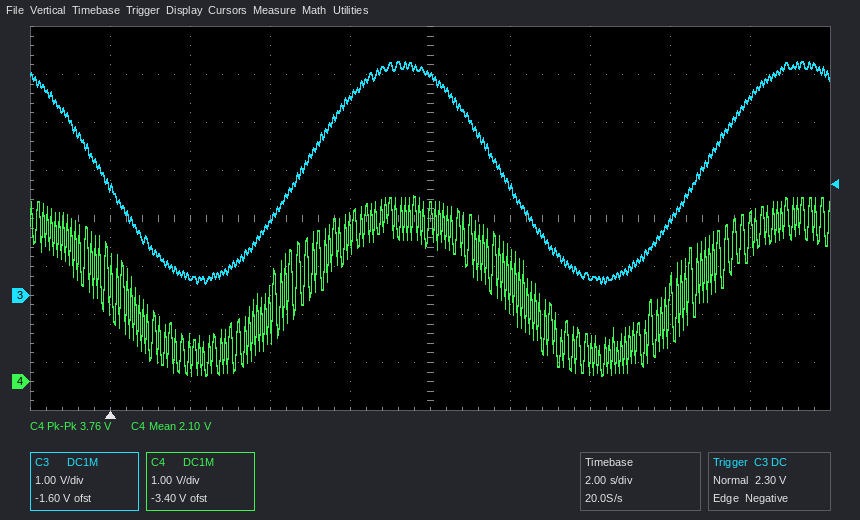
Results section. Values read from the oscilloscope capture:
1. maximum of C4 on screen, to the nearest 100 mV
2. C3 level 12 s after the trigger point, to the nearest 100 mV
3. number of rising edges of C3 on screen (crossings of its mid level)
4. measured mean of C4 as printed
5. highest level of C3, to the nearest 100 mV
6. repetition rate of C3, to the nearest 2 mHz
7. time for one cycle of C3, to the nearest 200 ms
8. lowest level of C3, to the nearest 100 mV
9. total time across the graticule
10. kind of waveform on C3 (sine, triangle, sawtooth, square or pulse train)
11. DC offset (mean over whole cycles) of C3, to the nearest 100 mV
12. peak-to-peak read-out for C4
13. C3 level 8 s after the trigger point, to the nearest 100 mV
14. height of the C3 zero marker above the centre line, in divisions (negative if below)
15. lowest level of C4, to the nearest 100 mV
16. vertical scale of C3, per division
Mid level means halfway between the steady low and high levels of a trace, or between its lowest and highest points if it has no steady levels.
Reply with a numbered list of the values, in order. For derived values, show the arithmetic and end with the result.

1. 3.9 V
2. 400 mV
3. 2
4. 2.10 V
5. 4.9 V
6. 1 / 10.0 s ≈ 100 mHz
7. 10.0 s
8. 200 mV
9. 20 s
10. sine
11. (4.9 V + (200 mV)) / 2 ≈ 2.6 V
12. 3.76 V
13. 4.6 V
14. -1.6 div
15. 100 mV
16. 1 V
